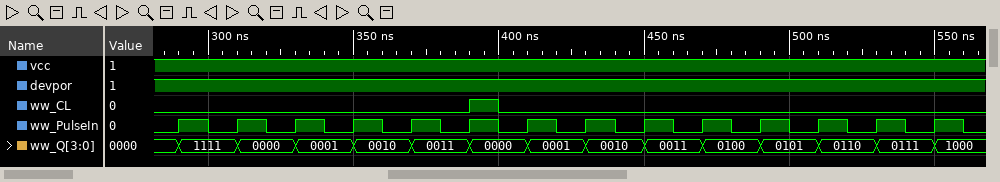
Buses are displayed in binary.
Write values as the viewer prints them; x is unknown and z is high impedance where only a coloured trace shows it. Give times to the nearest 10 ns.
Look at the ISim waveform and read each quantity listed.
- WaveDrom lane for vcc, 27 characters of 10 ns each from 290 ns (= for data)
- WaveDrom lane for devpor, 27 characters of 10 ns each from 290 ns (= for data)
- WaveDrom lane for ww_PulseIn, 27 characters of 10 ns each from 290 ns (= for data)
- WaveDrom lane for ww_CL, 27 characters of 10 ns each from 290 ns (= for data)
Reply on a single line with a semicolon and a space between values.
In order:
{name: 'vcc', wave: '1..........................'}; {name: 'devpor', wave: '1..........................'}; {name: 'ww_PulseIn', wave: '101010101010101010101010101'}; {name: 'ww_CL', wave: '0.........10...............'}
